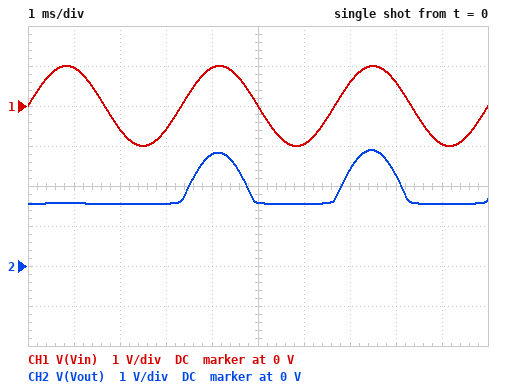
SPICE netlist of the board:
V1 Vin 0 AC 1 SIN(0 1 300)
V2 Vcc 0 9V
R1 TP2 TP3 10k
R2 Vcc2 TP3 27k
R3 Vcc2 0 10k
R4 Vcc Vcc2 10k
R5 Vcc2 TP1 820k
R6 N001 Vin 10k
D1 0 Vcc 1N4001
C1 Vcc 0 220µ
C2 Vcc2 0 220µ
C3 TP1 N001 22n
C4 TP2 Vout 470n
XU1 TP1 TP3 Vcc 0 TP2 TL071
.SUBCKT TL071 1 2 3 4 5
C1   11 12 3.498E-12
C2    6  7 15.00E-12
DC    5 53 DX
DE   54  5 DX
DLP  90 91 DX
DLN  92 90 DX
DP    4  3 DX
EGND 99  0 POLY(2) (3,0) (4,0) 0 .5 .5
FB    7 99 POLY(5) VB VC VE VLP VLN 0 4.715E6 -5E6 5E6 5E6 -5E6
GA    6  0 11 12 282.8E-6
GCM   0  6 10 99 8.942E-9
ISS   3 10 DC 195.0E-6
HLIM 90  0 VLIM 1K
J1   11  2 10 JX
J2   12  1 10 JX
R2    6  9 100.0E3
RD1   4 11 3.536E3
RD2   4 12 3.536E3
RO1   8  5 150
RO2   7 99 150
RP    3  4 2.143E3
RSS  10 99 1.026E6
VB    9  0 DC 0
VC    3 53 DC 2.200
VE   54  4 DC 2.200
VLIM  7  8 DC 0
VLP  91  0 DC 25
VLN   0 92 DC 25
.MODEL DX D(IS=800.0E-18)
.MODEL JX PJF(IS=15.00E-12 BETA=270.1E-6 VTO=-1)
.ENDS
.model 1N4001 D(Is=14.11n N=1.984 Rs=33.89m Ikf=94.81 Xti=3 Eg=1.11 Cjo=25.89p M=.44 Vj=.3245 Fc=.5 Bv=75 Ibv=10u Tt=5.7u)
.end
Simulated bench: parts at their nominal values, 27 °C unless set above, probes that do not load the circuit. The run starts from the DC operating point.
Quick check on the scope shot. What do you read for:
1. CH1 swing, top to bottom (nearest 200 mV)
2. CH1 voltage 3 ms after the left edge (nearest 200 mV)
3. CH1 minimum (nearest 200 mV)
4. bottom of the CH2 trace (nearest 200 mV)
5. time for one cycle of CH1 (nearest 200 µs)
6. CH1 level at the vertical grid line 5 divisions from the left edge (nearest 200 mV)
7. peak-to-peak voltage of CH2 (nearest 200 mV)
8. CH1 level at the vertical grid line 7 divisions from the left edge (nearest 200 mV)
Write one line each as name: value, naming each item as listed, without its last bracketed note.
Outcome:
CH1 swing, top to bottom: 2.0 V
CH1 voltage 3 ms after the left edge: -600 mV
CH1 minimum: -1.0 V
bottom of the CH2 trace: 1.6 V
time for one cycle of CH1: 3.4 ms
CH1 level at the vertical grid line 5 divisions from the left edge: 0 V
peak-to-peak voltage of CH2: 1.4 V
CH1 level at the vertical grid line 7 divisions from the left edge: 600 mV
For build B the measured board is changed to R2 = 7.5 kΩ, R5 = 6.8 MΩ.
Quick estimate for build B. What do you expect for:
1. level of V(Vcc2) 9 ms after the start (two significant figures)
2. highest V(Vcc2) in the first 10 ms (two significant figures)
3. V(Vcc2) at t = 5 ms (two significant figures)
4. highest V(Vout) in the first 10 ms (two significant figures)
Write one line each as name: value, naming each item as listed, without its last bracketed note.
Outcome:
level of V(Vcc2) 9 ms after the start: 43 mV
highest V(Vcc2) in the first 10 ms: 47 mV
V(Vcc2) at t = 5 ms: 24 mV
highest V(Vout) in the first 10 ms: 5.0 V
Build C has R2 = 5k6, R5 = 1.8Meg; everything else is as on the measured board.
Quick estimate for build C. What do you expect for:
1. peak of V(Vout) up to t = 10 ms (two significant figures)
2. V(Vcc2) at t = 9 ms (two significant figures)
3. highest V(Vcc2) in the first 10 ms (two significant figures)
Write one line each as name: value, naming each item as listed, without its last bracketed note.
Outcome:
peak of V(Vout) up to t = 10 ms: 5.8 V
V(Vcc2) at t = 9 ms: 44 mV
highest V(Vcc2) in the first 10 ms: 49 mV
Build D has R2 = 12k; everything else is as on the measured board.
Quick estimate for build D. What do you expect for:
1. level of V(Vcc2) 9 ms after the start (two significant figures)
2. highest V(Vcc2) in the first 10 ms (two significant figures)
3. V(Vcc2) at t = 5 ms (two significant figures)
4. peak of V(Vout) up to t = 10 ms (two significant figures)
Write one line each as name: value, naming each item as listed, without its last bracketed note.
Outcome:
level of V(Vcc2) 9 ms after the start: 41 mV
highest V(Vcc2) in the first 10 ms: 45 mV
V(Vcc2) at t = 5 ms: 23 mV
peak of V(Vout) up to t = 10 ms: 3.7 V
